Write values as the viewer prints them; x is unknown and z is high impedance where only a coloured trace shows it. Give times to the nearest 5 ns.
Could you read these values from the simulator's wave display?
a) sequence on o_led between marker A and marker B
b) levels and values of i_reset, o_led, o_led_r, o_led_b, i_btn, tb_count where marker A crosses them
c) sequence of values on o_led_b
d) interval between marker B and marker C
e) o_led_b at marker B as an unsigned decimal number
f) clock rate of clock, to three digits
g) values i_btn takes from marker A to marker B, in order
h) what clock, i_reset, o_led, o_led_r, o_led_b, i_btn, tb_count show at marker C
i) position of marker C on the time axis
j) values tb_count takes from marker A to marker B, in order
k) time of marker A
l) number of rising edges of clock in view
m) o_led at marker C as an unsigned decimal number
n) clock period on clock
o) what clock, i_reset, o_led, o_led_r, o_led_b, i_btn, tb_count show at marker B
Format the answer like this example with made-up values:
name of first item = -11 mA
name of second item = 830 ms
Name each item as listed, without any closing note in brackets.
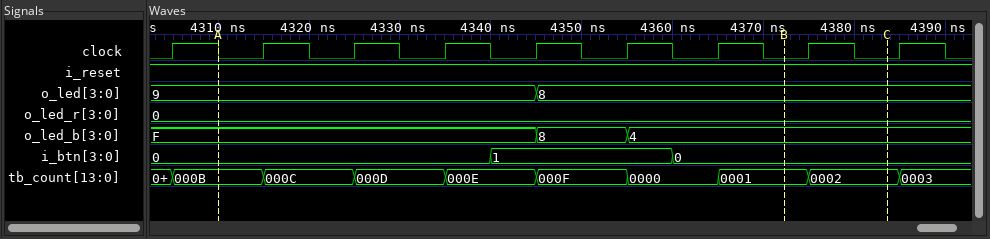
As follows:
sequence on o_led between marker A and marker B = 9, 8
levels and values of i_reset, o_led, o_led_r, o_led_b, i_btn, tb_count where marker A crosses them = i_reset=1, o_led=9, o_led_r=0, o_led_b=F, i_btn=0, tb_count=000B
sequence of values on o_led_b = F, 8, 4
interval between marker B and marker C = 10 ns
o_led_b at marker B as an unsigned decimal number = 4
clock rate of clock, to three digits = 100 MHz
values i_btn takes from marker A to marker B, in order = 0, 1, 0
what clock, i_reset, o_led, o_led_r, o_led_b, i_btn, tb_count show at marker C = clock=0, i_reset=1, o_led=8, o_led_r=0, o_led_b=4, i_btn=0, tb_count=0002
position of marker C on the time axis = 4385 ns
values tb_count takes from marker A to marker B, in order = 000B, 000C, 000D, 000E, 000F, 0000, 0001
time of marker A = 4310 ns
number of rising edges of clock in view = 9
o_led at marker C as an unsigned decimal number = 8
clock period on clock = 10 ns
what clock, i_reset, o_led, o_led_r, o_led_b, i_btn, tb_count show at marker B = clock=0, i_reset=1, o_led=8, o_led_r=0, o_led_b=4, i_btn=0, tb_count=0001
